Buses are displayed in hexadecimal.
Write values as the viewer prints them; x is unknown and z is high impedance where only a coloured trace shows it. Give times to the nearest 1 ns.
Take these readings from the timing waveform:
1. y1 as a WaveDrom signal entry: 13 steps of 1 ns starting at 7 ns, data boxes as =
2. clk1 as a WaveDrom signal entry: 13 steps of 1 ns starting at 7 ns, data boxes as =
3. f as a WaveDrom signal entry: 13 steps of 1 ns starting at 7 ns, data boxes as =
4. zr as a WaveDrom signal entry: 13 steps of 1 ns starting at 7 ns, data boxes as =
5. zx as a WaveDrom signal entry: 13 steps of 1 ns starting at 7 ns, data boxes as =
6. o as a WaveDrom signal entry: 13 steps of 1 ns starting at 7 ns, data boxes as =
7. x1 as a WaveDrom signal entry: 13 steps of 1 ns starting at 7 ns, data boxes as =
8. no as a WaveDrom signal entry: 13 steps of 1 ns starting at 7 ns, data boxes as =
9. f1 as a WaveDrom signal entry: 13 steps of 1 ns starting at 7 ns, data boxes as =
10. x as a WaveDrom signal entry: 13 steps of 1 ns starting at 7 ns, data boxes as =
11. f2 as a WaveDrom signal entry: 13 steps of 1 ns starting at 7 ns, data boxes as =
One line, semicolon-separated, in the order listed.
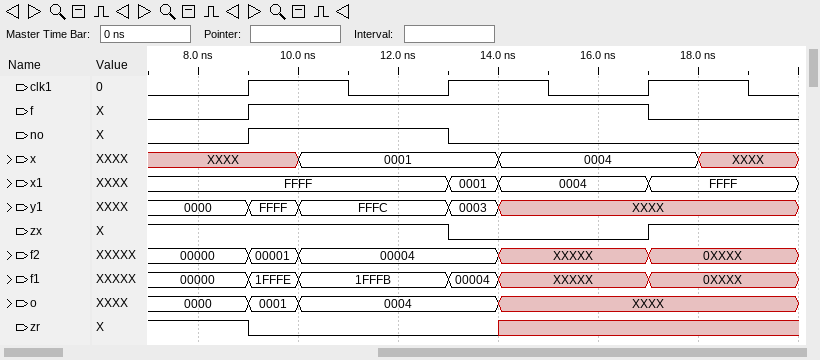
{name: 'y1', wave: '=.==..=x.....', data: '0000 FFFF FFFC 0003'}; {name: 'clk1', wave: '0.1.0.1.0.1.0'}; {name: 'f', wave: '0.1.......0..'}; {name: 'zr', wave: '1.0....x.....'}; {name: 'zx', wave: '1.....0...1..'}; {name: 'o', wave: '=.==...x.....', data: '0000 0001 0004'}; {name: 'x1', wave: '=.....==..=..', data: 'FFFF 0001 0004 FFFF'}; {name: 'no', wave: '0.1...0......'}; {name: 'f1', wave: '=.==..=x..=..', data: '00000 1FFFE 1FFFB 00004 0XXXX'}; {name: 'x', wave: 'x..=...=...x.', data: '0001 0004'}; {name: 'f2', wave: '=.==...x..=..', data: '00000 00001 00004 0XXXX'}
